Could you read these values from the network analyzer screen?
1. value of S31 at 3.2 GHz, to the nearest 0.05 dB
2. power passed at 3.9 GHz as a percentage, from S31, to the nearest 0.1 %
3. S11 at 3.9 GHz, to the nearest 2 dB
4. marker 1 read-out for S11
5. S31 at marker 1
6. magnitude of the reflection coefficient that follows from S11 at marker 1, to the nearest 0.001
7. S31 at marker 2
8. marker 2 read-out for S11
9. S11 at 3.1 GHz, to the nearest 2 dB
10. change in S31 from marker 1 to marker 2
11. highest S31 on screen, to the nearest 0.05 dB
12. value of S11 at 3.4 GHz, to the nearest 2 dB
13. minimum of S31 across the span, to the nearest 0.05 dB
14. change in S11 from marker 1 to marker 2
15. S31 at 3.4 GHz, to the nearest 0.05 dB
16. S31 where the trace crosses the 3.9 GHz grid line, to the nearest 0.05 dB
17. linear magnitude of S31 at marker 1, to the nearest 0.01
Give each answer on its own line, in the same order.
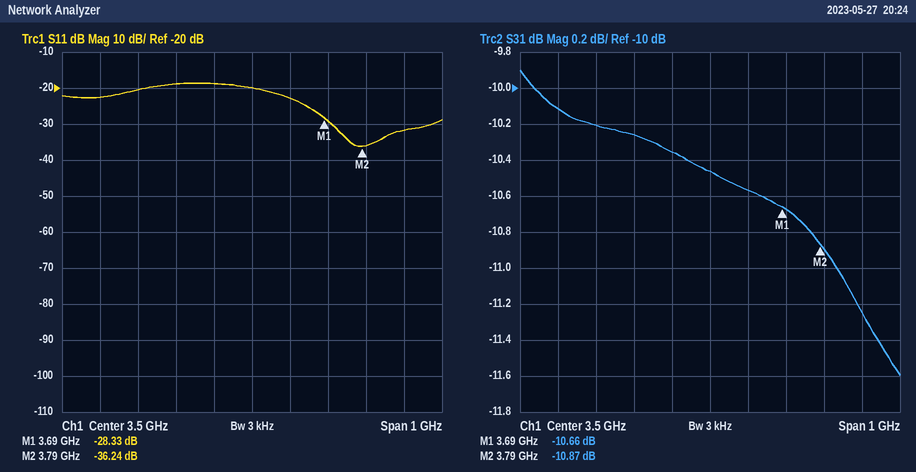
-10.20 dB
7.5 %
-32 dB
-28.33 dB
-10.66 dB
0.038
-10.87 dB
-36.24 dB
-22 dB
-0.21 dB
-9.90 dB
-18 dB
-11.60 dB
-7.91 dB
-10.35 dB
-11.25 dB
0.29
